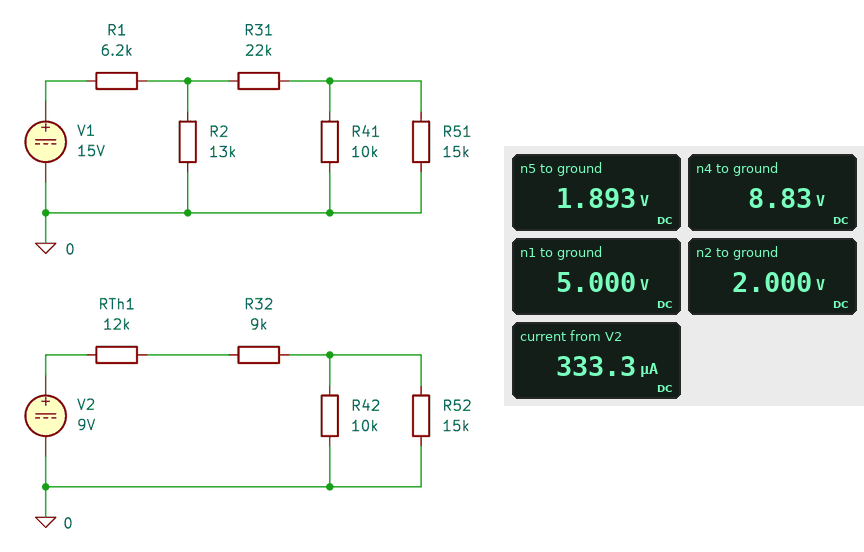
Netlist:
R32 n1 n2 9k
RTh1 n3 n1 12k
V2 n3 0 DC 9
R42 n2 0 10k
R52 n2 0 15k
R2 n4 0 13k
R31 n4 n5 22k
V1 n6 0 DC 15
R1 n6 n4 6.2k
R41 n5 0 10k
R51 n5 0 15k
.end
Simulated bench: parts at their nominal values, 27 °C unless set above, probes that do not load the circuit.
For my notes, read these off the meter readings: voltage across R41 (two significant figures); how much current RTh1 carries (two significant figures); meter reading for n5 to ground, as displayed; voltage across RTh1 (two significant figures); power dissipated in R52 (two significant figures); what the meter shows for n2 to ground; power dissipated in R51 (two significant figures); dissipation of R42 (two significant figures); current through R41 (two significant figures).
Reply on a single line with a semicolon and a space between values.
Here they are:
1.9 V; 330 µA; 1.893 V; 4.0 V; 270 µW; 2.000 V; 240 µW; 400 µW; 190 µA
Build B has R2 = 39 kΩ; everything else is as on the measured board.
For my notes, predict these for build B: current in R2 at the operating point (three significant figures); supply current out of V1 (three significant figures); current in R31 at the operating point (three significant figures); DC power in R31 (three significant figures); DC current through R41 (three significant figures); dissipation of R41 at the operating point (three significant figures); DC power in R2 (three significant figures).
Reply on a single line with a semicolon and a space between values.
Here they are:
279 µA; 667 µA; 388 µA; 3.31 mW; 233 µA; 542 µW; 3.03 mW
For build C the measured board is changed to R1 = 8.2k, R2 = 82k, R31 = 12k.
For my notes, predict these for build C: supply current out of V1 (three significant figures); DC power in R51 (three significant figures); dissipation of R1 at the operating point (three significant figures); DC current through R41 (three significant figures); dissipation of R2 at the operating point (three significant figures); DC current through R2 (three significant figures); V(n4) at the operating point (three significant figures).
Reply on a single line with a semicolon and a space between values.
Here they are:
653 µA; 689 µW; 3.50 mW; 321 µA; 1.13 mW; 118 µA; 9.64 V
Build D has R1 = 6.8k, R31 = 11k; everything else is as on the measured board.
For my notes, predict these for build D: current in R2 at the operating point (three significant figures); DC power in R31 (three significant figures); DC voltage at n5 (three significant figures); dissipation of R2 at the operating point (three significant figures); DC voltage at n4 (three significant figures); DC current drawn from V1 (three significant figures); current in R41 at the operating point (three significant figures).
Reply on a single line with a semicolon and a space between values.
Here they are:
600 µA; 2.32 mW; 2.75 V; 4.68 mW; 7.80 V; 1.06 mA; 275 µA
